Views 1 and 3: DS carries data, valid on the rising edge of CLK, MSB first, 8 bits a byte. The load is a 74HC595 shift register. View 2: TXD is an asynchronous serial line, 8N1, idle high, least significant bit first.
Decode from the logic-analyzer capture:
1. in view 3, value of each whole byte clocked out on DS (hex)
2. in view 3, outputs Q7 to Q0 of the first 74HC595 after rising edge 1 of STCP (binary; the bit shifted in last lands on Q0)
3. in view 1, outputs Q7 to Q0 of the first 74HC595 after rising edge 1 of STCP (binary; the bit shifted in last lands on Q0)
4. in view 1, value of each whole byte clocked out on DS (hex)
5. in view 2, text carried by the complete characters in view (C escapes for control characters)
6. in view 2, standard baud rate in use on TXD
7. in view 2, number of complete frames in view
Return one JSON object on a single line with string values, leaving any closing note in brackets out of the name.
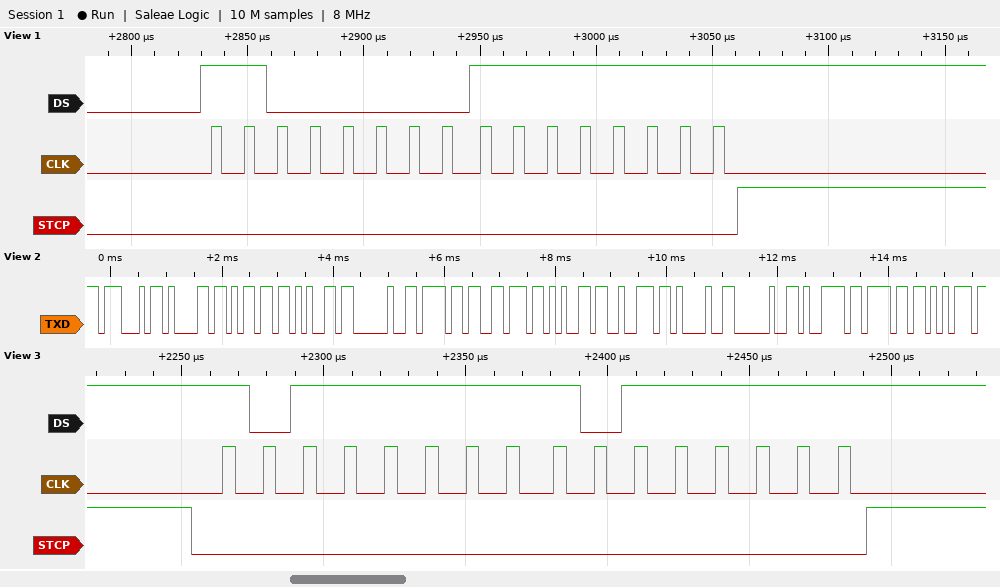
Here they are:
{"in view 3, value of each whole byte clocked out on DS": "0xBF 0xBF", "in view 3, outputs Q7 to Q0 of the first 74HC595 after rising edge 1 of STCP": "10111111", "in view 1, outputs Q7 to Q0 of the first 74HC595 after rising edge 1 of STCP": "11111111", "in view 1, value of each whole byte clocked out on DS": "C0 FF", "in view 2, text carried by the complete characters in view": "\"Game over! you\"", "in view 2, standard baud rate in use on TXD": "9600 baud", "in view 2, number of complete frames in view": "14"}
